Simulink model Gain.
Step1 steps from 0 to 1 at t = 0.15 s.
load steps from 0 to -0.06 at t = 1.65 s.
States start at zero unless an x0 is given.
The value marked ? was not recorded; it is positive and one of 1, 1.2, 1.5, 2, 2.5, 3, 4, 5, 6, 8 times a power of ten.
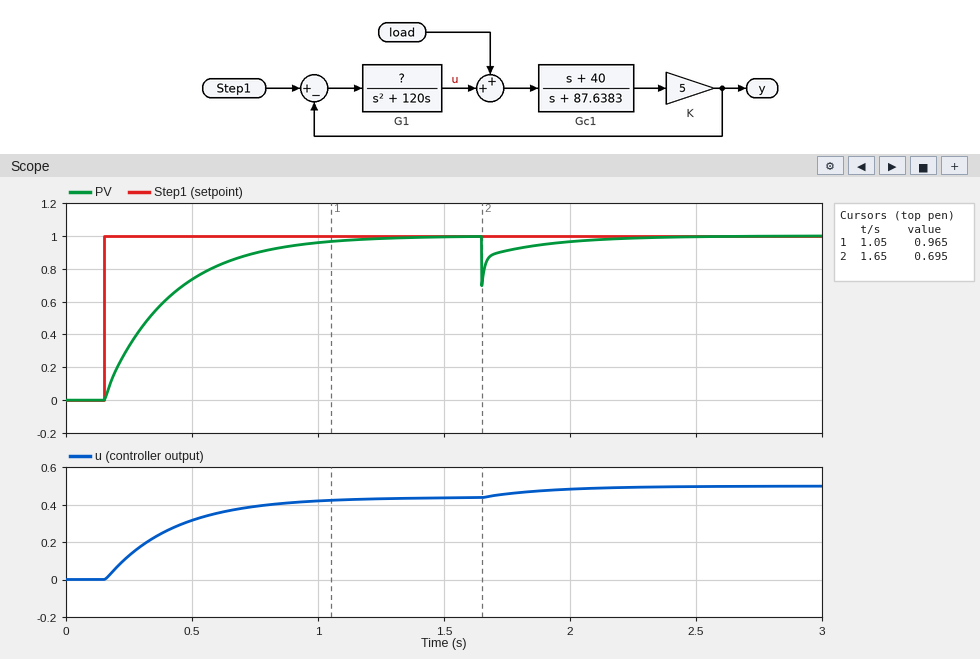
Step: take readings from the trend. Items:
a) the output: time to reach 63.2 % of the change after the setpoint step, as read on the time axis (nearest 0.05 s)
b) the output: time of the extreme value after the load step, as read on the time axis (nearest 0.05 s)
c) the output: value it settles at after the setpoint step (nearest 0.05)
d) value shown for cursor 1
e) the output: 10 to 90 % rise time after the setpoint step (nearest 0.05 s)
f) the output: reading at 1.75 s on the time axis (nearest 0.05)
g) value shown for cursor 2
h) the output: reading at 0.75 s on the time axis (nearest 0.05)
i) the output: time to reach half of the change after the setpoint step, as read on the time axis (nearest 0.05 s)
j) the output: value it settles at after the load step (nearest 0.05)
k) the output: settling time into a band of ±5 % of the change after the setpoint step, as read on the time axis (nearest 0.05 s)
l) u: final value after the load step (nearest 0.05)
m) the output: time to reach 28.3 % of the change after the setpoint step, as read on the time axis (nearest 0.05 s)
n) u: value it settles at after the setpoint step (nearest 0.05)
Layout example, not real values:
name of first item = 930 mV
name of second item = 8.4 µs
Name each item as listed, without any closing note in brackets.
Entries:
the output: time to reach 63.2 % of the change after the setpoint step, as read on the time axis = 0.40 s
the output: time of the extreme value after the load step, as read on the time axis = 1.65 s
the output: value it settles at after the setpoint step = 1.00
value shown for cursor 1 = 0.965
the output: 10 to 90 % rise time after the setpoint step = 0.60 s
the output: reading at 1.75 s on the time axis = 0.90
value shown for cursor 2 = 0.695
the output: reading at 0.75 s on the time axis = 0.90
the output: time to reach half of the change after the setpoint step, as read on the time axis = 0.35 s
the output: value it settles at after the load step = 1.00
the output: settling time into a band of ±5 % of the change after the setpoint step, as read on the time axis = 0.95 s
u: final value after the load step = 0.50
the output: time to reach 28.3 % of the change after the setpoint step, as read on the time axis = 0.25 s
u: value it settles at after the setpoint step = 0.45
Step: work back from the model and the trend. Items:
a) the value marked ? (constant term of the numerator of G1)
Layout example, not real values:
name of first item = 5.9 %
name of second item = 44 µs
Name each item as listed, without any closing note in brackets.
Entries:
the value marked ? = 200
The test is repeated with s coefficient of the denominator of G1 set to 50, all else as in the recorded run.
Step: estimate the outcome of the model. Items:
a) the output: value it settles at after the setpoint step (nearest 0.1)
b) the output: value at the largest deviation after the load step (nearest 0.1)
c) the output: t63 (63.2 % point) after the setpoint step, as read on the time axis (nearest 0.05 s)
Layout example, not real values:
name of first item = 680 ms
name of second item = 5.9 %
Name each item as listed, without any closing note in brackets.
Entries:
the output: value it settles at after the setpoint step = 1.0
the output: value at the largest deviation after the load step = 0.7
the output: t63 (63.2 % point) after the setpoint step, as read on the time axis = 0.25 s
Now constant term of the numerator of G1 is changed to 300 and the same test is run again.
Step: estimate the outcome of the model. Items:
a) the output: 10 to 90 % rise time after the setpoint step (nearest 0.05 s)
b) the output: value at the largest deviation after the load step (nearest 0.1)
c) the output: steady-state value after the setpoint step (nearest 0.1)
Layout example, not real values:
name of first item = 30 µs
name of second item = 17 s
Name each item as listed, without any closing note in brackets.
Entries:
the output: 10 to 90 % rise time after the setpoint step = 0.40 s
the output: value at the largest deviation after the load step = 0.7
the output: steady-state value after the setpoint step = 1.0
